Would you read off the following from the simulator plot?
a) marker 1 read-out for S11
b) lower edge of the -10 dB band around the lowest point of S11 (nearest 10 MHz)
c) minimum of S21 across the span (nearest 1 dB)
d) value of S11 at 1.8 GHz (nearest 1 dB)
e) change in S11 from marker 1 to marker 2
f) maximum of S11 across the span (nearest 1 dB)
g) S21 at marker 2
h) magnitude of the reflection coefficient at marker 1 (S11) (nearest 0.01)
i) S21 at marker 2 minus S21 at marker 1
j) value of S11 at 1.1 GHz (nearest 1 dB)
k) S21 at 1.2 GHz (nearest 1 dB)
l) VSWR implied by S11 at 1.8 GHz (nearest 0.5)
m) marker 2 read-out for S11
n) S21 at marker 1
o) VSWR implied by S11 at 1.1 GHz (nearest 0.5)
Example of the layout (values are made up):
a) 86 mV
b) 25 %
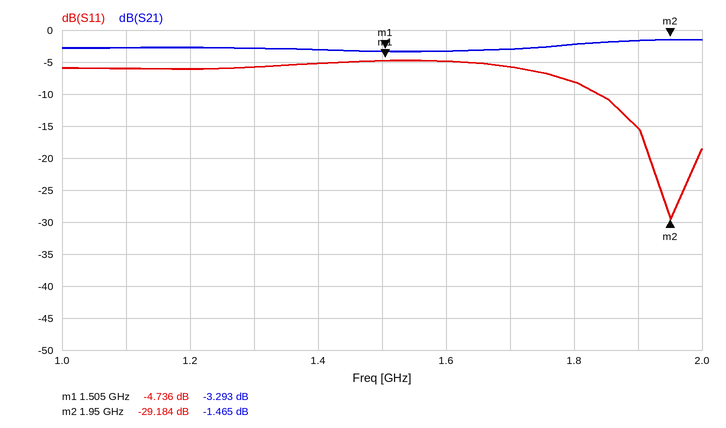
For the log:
a) -4.736 dB
b) 1.84 GHz
c) -3 dB
d) -8 dB
e) -24.448 dB
f) -5 dB
g) -1.465 dB
h) 0.58
i) 1.828 dB
j) -6 dB
k) -3 dB
l) 2.5
m) -29.184 dB
n) -3.293 dB
o) 3.0
